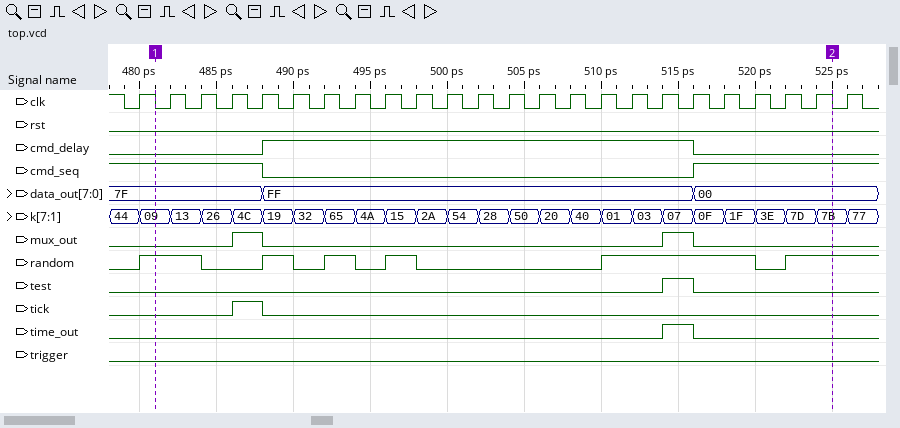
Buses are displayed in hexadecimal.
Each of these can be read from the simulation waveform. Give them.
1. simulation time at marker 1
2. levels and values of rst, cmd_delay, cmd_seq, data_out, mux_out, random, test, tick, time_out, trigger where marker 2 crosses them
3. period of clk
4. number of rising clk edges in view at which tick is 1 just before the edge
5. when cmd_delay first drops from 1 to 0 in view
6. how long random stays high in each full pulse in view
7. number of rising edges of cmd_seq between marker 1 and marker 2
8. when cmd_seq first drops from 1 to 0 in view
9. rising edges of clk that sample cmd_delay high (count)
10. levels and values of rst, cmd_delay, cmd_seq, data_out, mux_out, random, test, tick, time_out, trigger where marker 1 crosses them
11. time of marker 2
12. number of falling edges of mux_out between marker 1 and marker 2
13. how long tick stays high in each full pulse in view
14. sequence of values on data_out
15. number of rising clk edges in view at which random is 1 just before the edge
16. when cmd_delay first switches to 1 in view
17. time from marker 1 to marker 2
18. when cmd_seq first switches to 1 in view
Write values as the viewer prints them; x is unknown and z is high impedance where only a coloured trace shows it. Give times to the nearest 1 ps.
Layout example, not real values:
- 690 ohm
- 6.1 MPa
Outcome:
- 481 ps
- rst=0, cmd_delay=0, cmd_seq=1, data_out=00, mux_out=0, random=1, test=0, tick=0, time_out=0, trigger=0
- 2 ps
- 1
- 516 ps
- 4 ps, 2 ps, 2 ps, 2 ps, 10 ps
- 1
- 488 ps
- 14
- rst=0, cmd_delay=0, cmd_seq=1, data_out=7F, mux_out=0, random=1, test=0, tick=0, time_out=0, trigger=0
- 525 ps
- 2
- 2 ps
- 7F, FF, 00
- 12
- 488 ps
- 44 ps
- 516 ps
